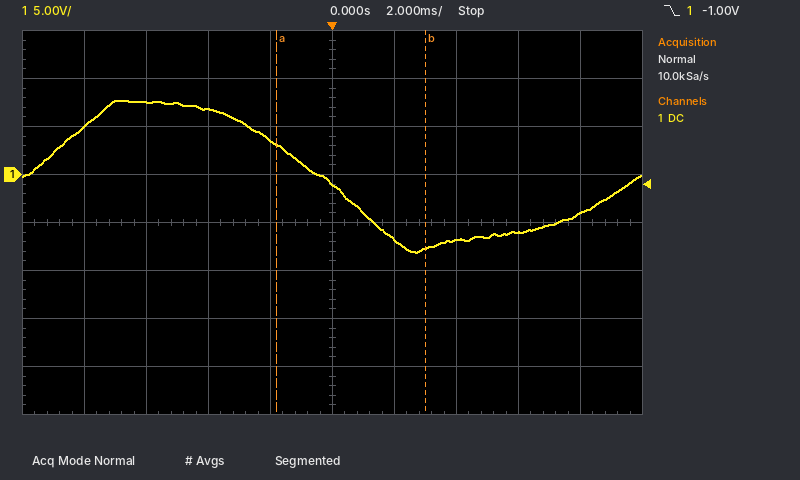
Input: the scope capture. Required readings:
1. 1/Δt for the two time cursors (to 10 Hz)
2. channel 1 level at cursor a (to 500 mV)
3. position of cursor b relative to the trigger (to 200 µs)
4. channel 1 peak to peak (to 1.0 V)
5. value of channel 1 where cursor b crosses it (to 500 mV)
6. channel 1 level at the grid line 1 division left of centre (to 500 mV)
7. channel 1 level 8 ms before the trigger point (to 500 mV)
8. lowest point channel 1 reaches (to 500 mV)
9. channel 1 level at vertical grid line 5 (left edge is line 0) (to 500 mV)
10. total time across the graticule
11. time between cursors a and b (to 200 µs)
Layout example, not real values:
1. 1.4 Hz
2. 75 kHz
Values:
1. 210 Hz
2. 3.0 V
3. +3.0 ms
4. 16.0 V
5. -7.5 V
6. 3.5 V
7. 5.0 V
8. -8.0 V
9. -1.0 V
10. 20 ms
11. 4.8 ms
